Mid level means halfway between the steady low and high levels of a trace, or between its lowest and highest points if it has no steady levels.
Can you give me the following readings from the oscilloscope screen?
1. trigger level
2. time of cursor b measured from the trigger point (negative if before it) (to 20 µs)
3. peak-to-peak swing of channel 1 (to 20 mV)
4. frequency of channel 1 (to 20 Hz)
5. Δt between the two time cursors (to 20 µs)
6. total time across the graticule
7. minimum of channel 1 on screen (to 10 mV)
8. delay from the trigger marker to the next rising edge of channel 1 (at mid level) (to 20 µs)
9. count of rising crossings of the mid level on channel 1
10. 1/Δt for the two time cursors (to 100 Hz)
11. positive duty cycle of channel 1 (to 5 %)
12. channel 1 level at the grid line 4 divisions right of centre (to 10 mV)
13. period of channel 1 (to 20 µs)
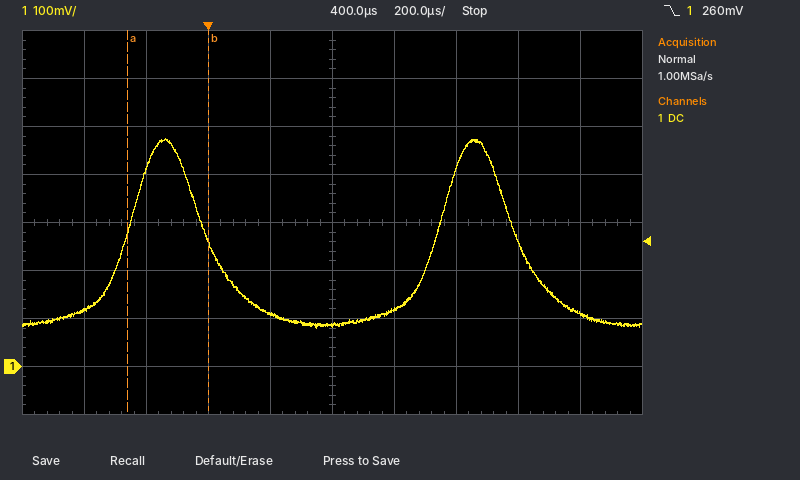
260 mV
0 µs
400 mV
1.00 kHz
260 µs
2 ms
80 mV
740 µs
2
3.8 kHz
25 %
110 mV
1.00 ms
